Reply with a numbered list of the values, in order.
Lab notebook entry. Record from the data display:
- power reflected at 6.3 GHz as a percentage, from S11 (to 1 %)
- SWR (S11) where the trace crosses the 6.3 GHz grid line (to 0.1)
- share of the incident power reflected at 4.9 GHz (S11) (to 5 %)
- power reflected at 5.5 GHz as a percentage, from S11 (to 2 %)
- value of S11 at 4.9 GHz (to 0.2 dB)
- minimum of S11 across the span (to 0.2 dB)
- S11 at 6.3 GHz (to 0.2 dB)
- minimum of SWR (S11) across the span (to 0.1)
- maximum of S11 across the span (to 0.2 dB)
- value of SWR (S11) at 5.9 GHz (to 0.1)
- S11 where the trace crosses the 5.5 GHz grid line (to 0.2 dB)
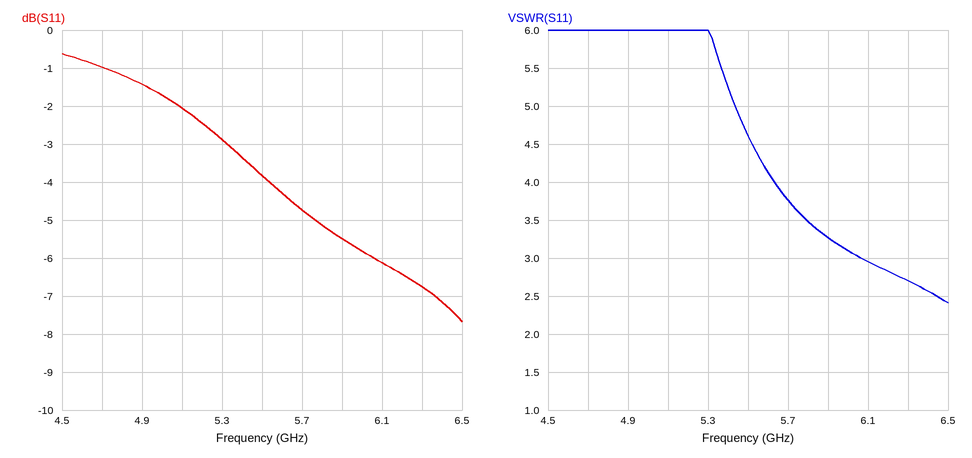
1. 21 %
2. 2.7
3. 70 %
4. 42 %
5. -1.4 dB
6. -7.6 dB
7. -6.8 dB
8. 2.4
9. -0.6 dB
10. 3.3
11. -3.8 dB
